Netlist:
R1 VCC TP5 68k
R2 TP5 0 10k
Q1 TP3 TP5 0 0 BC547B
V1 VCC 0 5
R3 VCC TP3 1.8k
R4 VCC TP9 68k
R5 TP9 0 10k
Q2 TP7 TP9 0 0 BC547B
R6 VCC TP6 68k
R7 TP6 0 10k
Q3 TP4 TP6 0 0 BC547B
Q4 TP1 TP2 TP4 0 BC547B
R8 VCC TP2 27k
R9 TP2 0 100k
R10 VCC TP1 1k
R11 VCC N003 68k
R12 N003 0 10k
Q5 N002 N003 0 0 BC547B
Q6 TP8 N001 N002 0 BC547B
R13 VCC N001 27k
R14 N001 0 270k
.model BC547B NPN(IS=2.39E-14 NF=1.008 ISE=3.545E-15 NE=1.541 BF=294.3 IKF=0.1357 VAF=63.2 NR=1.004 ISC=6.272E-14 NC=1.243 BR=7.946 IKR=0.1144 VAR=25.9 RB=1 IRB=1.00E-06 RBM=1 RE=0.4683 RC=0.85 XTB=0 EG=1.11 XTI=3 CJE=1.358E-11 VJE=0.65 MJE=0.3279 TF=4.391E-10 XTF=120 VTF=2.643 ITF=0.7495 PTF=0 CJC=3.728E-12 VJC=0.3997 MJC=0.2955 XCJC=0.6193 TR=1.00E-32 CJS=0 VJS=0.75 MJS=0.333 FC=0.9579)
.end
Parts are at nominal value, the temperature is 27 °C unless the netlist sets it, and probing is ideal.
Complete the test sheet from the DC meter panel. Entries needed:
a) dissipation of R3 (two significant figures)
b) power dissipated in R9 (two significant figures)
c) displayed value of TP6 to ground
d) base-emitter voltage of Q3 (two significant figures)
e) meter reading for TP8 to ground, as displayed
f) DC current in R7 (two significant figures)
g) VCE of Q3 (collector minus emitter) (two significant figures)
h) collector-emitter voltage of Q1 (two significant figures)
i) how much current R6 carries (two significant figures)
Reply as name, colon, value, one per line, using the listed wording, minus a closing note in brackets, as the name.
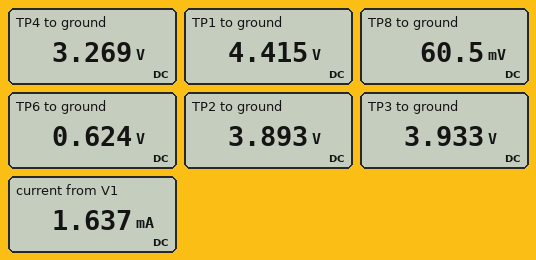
dissipation of R3: 630 µW
power dissipated in R9: 150 µW
displayed value of TP6 to ground: 0.624 V
base-emitter voltage of Q3: 620 mV
meter reading for TP8 to ground, as displayed: 60.5 mV
DC current in R7: 62 µA
VCE of Q3 (collector minus emitter): 3.3 V
collector-emitter voltage of Q1: 3.9 V
how much current R6 carries: 64 µA
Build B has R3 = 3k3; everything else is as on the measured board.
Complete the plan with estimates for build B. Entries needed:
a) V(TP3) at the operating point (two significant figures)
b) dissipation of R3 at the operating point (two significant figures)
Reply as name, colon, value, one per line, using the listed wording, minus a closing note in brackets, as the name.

V(TP3) at the operating point: 3.1 V
dissipation of R3 at the operating point: 1.1 mW
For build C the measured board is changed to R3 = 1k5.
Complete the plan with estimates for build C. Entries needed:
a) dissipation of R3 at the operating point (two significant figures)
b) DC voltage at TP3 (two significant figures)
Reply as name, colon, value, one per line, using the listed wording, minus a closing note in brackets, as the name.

dissipation of R3 at the operating point: 530 µW
DC voltage at TP3: 4.1 V
